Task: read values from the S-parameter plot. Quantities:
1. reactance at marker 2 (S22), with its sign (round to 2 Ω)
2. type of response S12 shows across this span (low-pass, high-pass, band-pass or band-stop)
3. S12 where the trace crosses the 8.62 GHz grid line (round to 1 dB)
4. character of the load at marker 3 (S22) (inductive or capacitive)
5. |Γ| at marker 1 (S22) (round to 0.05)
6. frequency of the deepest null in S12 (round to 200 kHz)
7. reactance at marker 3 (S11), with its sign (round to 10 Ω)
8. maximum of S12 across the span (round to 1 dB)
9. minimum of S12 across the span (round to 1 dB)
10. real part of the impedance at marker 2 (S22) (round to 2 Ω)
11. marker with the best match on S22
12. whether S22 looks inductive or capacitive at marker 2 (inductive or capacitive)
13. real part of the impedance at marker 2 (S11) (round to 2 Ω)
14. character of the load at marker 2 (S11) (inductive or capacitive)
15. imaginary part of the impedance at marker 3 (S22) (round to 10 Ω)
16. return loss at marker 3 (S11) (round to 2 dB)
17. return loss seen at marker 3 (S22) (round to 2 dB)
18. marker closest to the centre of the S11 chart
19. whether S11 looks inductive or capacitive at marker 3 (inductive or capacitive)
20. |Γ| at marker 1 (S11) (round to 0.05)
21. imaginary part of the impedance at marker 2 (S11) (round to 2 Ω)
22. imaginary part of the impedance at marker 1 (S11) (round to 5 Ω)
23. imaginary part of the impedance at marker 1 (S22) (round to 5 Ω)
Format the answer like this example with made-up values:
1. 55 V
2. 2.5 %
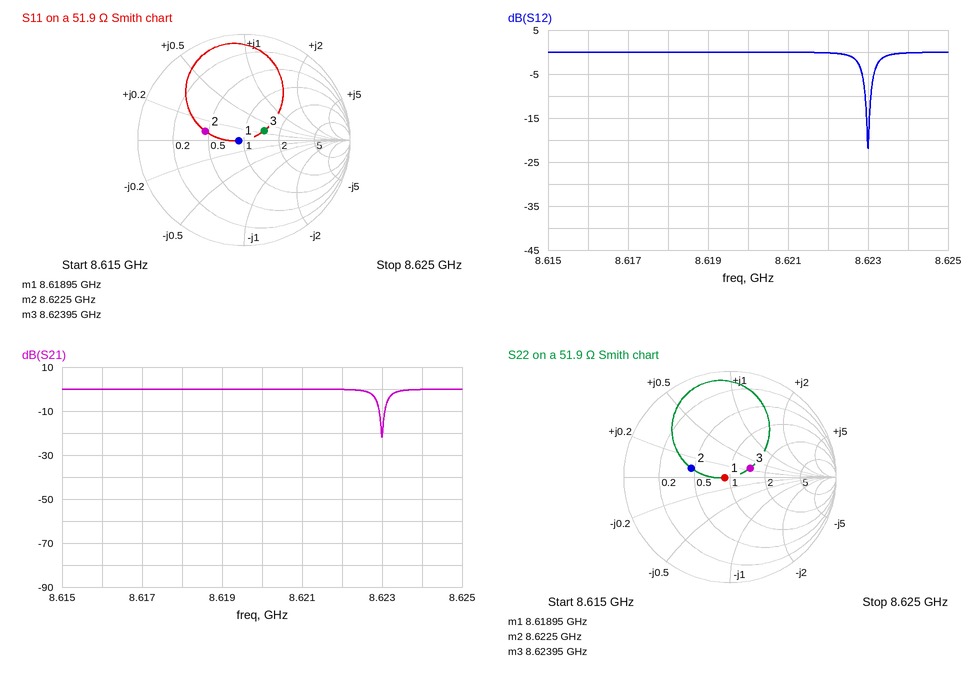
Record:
1. +4 Ω
2. band-stop
3. 0 dB
4. inductive
5. 0.05
6. 8.6230 GHz
7. +10 Ω
8. 0 dB
9. -22 dB
10. 24 Ω
11. marker 1
12. inductive
13. 24 Ω
14. inductive
15. +10 Ω
16. 14 dB
17. 14 dB
18. marker 1
19. inductive
20. 0.05
21. +4 Ω
22. 0 Ω
23. 0 Ω
